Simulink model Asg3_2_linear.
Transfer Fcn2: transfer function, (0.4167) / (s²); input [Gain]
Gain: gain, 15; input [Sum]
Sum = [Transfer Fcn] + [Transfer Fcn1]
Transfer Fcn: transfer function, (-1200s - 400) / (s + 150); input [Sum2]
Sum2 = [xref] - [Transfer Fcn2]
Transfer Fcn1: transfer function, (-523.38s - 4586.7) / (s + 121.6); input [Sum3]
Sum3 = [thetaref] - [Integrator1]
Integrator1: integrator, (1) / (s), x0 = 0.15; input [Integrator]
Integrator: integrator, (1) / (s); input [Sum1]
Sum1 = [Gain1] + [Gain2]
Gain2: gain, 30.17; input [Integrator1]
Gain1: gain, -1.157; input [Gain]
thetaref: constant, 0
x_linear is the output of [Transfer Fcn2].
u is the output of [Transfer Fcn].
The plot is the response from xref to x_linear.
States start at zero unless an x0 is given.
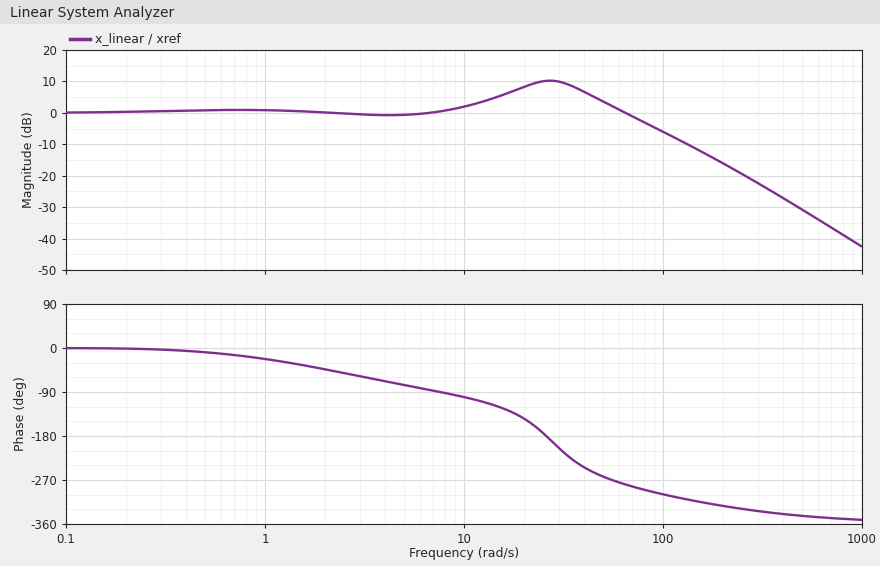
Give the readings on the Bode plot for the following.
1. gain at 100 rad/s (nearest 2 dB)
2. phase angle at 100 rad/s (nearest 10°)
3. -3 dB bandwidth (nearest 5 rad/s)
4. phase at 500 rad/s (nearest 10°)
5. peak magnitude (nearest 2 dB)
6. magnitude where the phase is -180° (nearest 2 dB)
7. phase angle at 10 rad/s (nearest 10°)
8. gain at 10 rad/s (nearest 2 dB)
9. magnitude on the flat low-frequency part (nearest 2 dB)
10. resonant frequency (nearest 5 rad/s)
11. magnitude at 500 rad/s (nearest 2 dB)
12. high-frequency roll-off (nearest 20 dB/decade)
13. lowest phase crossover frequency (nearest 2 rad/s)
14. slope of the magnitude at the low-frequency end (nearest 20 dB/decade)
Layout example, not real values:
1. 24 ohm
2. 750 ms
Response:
1. -6 dB
2. -300°
3. 80 rad/s
4. -340°
5. 10 dB
6. 10 dB
7. -100°
8. 2 dB
9. 0 dB
10. 25 rad/s
11. -30 dB
12. -40 dB/decade
13. 26 rad/s
14. 0 dB/decade
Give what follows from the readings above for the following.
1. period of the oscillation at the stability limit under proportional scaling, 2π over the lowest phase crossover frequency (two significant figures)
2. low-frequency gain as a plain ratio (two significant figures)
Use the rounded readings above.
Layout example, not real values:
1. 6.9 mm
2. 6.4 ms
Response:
1. 0.24 s
2. 1.0
